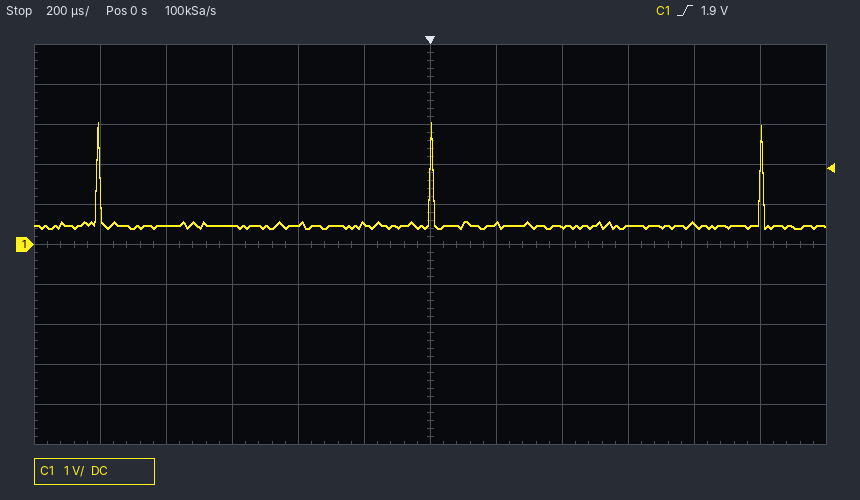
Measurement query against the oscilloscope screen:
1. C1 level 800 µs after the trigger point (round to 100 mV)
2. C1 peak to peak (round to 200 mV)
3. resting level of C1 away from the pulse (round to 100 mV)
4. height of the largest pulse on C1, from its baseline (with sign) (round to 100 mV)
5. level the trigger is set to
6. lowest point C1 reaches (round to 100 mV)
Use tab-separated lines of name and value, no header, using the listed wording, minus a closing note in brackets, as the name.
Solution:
C1 level 800 µs after the trigger point	500 mV
C1 peak to peak	2.6 V
resting level of C1 away from the pulse	500 mV
height of the largest pulse on C1, from its baseline (with sign)	+2.6 V
level the trigger is set to	1.9 V
lowest point C1 reaches	400 mV
